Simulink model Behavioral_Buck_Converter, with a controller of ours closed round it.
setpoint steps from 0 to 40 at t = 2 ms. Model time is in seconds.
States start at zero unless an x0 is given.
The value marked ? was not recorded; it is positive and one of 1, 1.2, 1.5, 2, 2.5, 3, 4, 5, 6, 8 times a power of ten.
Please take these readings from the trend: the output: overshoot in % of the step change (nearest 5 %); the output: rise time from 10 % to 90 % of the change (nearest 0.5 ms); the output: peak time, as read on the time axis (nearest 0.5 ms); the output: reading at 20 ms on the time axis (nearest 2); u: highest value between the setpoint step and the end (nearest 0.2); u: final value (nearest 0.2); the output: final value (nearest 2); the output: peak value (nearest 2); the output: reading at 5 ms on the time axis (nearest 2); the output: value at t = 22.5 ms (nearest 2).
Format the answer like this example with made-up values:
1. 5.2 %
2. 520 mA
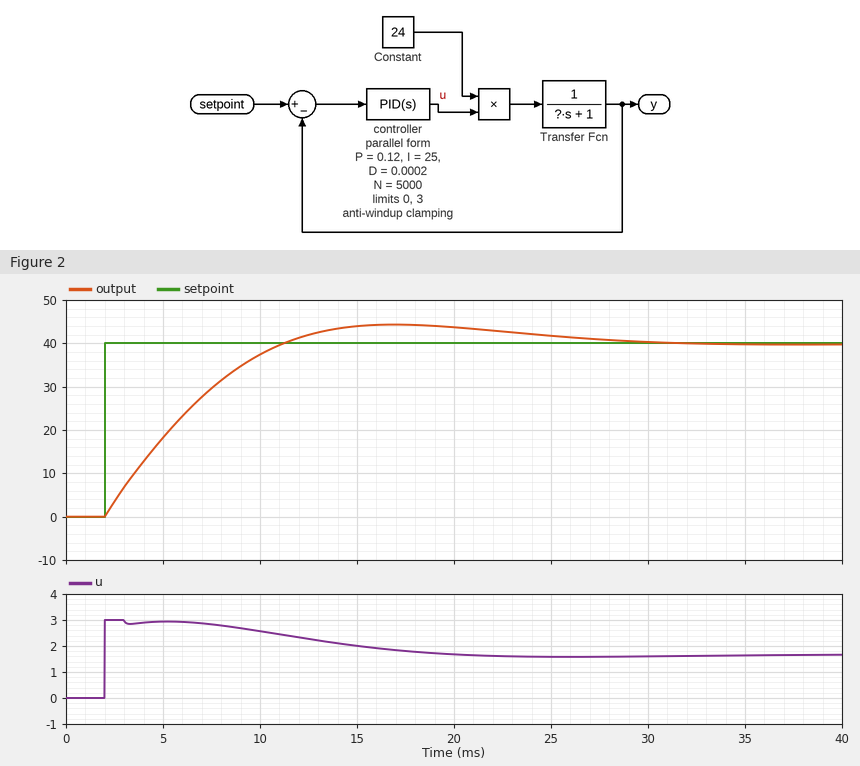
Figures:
1. 10 %
2. 7.0 ms
3. 17.0 ms
4. 44
5. 3.0
6. 1.6
7. 40
8. 44
9. 18
10. 42
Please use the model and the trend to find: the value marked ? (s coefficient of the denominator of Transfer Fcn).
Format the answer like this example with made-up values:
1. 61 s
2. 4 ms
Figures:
1. 0.01
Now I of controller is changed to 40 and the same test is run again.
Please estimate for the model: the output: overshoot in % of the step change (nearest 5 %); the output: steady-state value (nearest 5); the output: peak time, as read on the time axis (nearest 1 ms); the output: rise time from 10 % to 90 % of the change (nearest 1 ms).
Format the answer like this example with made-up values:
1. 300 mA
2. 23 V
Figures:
1. 15 %
2. 40
3. 15 ms
4. 6 ms
